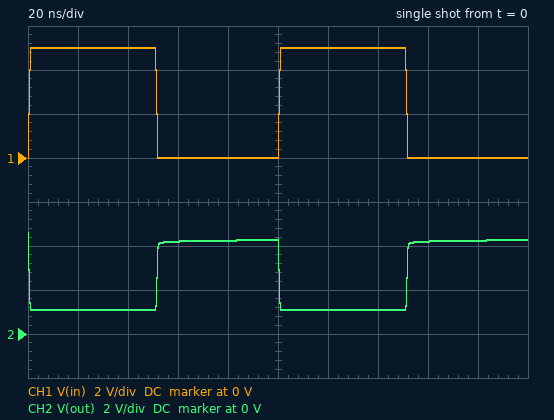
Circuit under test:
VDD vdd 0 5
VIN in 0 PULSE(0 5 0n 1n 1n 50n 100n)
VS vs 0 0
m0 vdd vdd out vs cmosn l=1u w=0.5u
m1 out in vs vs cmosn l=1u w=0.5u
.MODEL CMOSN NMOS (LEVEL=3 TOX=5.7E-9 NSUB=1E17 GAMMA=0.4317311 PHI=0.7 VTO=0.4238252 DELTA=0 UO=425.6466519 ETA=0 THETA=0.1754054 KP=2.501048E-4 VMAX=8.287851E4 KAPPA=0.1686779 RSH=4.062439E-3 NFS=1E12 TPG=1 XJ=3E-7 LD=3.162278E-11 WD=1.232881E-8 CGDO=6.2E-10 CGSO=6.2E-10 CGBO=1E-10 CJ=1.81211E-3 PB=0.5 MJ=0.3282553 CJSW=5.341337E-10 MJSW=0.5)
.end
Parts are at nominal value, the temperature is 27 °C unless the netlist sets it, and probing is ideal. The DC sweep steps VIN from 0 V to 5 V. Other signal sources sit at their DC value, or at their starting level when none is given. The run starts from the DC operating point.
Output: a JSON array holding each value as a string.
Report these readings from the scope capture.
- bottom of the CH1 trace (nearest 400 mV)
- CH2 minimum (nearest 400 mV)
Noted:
["0 V", "1.2 V"]
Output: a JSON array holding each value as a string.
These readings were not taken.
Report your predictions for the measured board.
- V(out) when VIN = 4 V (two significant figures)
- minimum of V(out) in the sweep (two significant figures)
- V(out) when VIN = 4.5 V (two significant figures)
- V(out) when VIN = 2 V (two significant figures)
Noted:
["1.3 V", "1.1 V", "1.2 V", "2.7 V"]
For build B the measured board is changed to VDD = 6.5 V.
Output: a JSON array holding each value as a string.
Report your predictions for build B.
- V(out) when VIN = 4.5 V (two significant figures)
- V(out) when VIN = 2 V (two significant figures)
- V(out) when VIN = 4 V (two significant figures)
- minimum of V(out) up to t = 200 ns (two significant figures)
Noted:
["2.0 V", "4.1 V", "2.4 V", "1.8 V"]
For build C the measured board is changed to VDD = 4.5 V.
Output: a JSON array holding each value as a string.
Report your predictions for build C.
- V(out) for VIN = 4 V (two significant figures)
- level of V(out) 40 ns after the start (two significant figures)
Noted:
["1.1 V", "890 mV"]
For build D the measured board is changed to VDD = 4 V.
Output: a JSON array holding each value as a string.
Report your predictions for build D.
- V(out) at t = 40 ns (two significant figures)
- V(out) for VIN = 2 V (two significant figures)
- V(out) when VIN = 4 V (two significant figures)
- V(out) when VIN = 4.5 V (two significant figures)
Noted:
["720 mV", "1.8 V", "850 mV", "780 mV"]
